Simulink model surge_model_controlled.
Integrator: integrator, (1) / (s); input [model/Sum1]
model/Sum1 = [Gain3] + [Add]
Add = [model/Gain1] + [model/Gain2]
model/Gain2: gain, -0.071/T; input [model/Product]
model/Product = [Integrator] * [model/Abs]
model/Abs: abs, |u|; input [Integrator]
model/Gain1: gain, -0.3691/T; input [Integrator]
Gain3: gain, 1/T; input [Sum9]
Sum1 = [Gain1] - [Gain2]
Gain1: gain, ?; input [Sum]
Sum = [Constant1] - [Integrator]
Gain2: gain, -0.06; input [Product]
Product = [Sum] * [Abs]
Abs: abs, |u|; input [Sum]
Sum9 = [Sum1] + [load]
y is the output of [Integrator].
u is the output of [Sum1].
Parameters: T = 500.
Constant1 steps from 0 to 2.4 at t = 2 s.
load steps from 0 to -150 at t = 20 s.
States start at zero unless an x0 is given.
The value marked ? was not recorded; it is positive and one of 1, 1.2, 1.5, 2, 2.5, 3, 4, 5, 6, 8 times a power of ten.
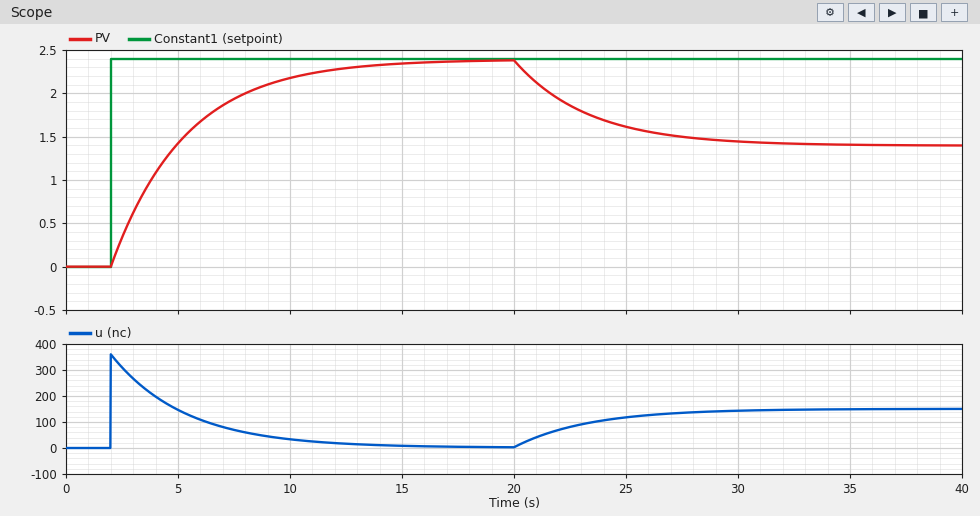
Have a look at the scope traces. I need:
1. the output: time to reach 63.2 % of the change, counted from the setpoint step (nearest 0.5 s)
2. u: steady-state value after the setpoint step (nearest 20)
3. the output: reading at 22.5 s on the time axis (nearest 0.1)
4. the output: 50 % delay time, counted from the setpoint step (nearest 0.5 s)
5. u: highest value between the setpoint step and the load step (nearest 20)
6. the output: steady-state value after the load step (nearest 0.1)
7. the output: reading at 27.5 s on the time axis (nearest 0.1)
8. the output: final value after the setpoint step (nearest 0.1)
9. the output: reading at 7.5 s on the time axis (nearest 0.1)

3.5 s
0
1.9
2.5 s
360
1.4
1.5
2.4
1.9
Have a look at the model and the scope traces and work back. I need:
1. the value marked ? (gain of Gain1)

150
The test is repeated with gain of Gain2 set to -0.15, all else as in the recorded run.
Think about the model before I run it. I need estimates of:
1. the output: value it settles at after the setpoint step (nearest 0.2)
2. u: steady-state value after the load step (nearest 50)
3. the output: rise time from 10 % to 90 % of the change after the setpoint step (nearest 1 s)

2.4
150
7 s
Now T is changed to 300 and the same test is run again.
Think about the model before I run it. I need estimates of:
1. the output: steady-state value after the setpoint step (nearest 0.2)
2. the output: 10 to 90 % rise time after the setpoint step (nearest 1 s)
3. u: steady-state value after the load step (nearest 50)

2.4
4 s
150
